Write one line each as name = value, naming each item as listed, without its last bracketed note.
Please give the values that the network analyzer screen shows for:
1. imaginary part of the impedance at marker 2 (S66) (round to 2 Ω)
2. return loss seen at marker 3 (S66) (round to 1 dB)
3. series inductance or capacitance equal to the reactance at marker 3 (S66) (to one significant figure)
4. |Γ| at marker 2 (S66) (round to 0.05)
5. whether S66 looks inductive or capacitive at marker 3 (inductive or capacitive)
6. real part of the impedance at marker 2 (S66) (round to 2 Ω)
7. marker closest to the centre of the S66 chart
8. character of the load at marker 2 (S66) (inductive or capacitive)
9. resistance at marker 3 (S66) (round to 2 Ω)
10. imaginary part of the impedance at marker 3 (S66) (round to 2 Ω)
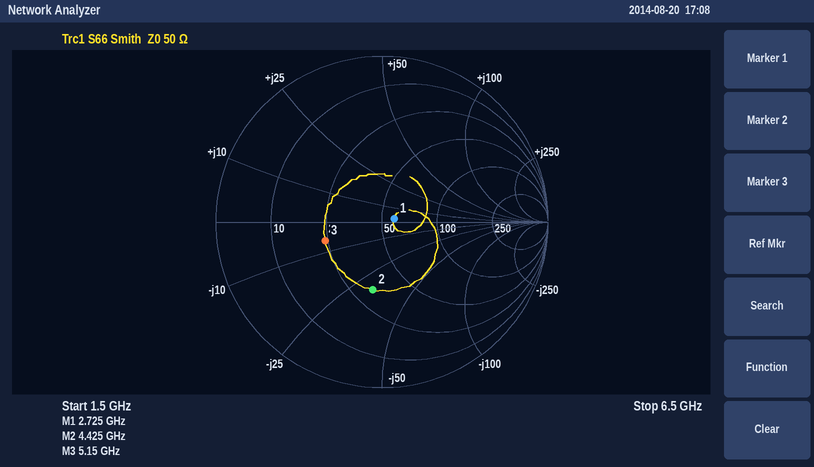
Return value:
imaginary part of the impedance at marker 2 (S66) = -32 Ω
return loss seen at marker 3 (S66) = 9 dB
series inductance or capacitance equal to the reactance at marker 3 (S66) = 5 pF
|Γ| at marker 2 (S66) = 0.40
whether S66 looks inductive or capacitive at marker 3 = capacitive
real part of the impedance at marker 2 (S66) = 32 Ω
marker closest to the centre of the S66 chart = marker 1
character of the load at marker 2 (S66) = capacitive
resistance at marker 3 (S66) = 24 Ω
imaginary part of the impedance at marker 3 (S66) = -6 Ω
